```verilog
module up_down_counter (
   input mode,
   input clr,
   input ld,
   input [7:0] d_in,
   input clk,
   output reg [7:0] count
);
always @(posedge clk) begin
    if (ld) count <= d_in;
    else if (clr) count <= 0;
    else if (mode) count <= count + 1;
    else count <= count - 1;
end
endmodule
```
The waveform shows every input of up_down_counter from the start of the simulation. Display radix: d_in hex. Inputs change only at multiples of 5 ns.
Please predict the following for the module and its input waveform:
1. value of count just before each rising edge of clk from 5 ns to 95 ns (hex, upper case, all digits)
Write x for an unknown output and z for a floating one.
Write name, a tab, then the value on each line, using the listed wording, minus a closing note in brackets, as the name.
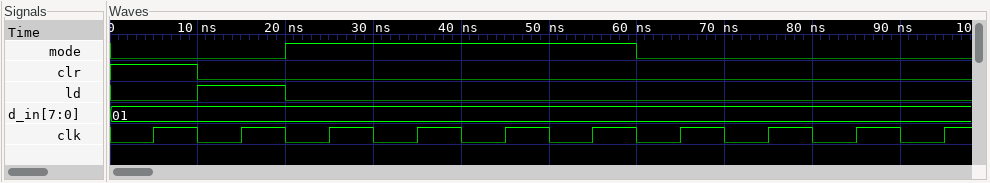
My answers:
value of count just before each rising edge of clk from 5 ns to 95 ns	x, 00, 01, 02, 03, 04, 05, 04, 03, 02
